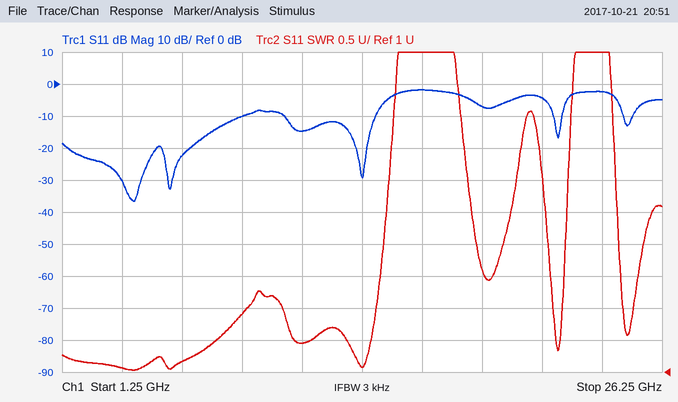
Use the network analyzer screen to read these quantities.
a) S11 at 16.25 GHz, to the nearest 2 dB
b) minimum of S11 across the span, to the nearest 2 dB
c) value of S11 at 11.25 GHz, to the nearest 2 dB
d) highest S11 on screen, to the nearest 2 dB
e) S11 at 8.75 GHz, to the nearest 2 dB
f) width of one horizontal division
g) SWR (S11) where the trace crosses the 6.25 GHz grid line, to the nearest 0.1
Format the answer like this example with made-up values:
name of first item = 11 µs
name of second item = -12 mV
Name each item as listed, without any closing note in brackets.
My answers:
S11 at 16.25 GHz, to the nearest 2 dB = -2 dB
minimum of S11 across the span, to the nearest 2 dB = -36 dB
value of S11 at 11.25 GHz, to the nearest 2 dB = -14 dB
highest S11 on screen, to the nearest 2 dB = -2 dB
S11 at 8.75 GHz, to the nearest 2 dB = -10 dB
width of one horizontal division = 2.5 GHz
SWR (S11) where the trace crosses the 6.25 GHz grid line, to the nearest 0.1 = 1.2
